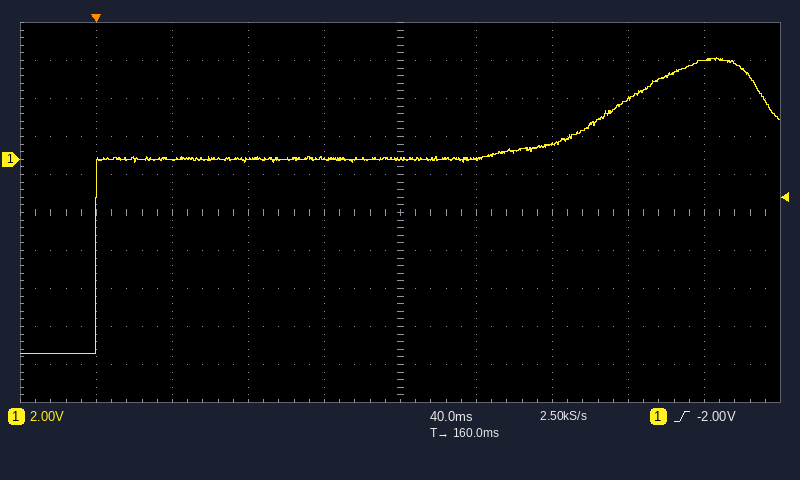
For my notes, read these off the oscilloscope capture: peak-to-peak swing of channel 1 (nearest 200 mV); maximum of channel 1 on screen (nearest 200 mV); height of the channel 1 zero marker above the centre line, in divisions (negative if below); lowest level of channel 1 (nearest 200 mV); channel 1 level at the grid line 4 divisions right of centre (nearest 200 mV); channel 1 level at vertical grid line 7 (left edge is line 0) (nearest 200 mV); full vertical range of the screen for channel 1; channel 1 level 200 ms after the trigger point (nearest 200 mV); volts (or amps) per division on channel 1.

15.6 V
5.4 V
+1.4 div
-10.2 V
5.2 V
800 mV
20 V
0.0 V
2 V
